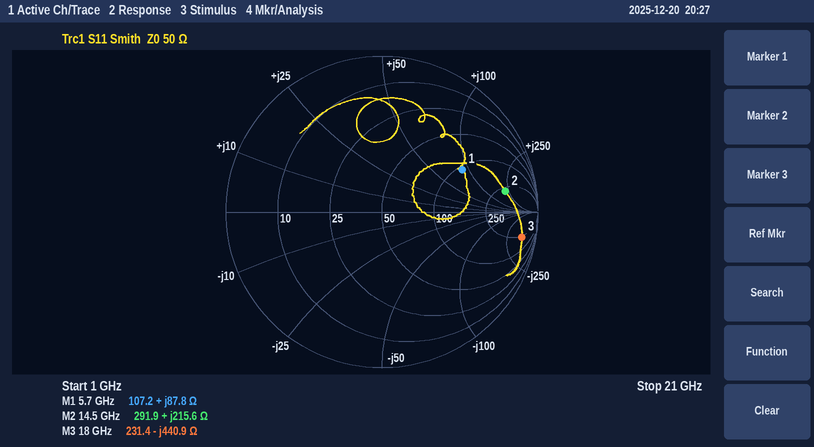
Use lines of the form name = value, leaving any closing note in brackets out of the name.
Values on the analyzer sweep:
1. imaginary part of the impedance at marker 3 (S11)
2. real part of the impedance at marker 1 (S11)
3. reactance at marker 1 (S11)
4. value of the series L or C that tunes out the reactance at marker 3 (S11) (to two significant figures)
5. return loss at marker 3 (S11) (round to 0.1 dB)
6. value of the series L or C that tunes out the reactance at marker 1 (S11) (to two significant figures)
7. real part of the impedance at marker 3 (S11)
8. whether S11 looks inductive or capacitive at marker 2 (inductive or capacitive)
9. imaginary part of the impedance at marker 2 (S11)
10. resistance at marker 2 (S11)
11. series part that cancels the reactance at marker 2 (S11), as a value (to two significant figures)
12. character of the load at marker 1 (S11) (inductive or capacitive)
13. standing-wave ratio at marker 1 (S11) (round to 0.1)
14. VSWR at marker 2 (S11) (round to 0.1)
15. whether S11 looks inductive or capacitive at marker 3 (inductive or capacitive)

imaginary part of the impedance at marker 3 = -440.9 Ω
real part of the impedance at marker 1 = 107.2 Ω
reactance at marker 1 = +87.8 Ω
value of the series L or C that tunes out the reactance at marker 3 (S11) = 3.9 nH
return loss at marker 3 (S11) = 0.8 dB
value of the series L or C that tunes out the reactance at marker 1 (S11) = 320 fF
real part of the impedance at marker 3 = 231.4 Ω
whether S11 looks inductive or capacitive at marker 2 = inductive
imaginary part of the impedance at marker 2 = +215.6 Ω
resistance at marker 2 = 291.9 Ω
series part that cancels the reactance at marker 2 (S11), as a value = 51 fF
character of the load at marker 1 (S11) = inductive
standing-wave ratio at marker 1 (S11) = 3.8
VSWR at marker 2 (S11) = 9.1
whether S11 looks inductive or capacitive at marker 3 = capacitive
